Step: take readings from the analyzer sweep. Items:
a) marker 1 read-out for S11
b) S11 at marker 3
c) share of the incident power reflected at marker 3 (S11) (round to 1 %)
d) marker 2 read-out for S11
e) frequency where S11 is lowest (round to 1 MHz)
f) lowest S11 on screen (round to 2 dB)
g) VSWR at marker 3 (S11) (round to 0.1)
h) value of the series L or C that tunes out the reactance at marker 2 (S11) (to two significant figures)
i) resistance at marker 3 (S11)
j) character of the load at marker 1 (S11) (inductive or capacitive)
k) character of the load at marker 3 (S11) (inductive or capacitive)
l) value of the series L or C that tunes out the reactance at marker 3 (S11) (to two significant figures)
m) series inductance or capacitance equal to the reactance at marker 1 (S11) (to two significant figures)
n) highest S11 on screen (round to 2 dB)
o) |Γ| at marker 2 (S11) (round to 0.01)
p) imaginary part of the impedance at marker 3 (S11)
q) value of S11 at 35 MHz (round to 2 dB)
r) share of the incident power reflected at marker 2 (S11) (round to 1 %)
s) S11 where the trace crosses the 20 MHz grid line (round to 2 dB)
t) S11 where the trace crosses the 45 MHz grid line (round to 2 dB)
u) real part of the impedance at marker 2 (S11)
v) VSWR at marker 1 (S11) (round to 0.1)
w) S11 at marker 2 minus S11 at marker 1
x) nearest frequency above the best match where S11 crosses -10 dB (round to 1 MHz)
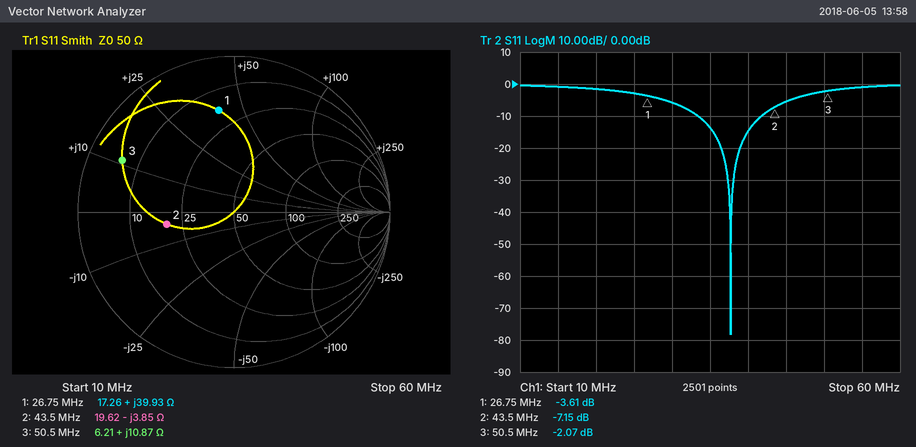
-3.61 dB
-2.07 dB
62 %
-7.15 dB
38 MHz
-78 dB
8.4
14 nH
6.21 Ω
inductive
inductive
290 pF
240 nH
0 dB
0.44
+10.87 Ω
-14 dB
19 %
-2 dB
-6 dB
19.62 Ω
4.9
-3.54 dB
42 MHz
